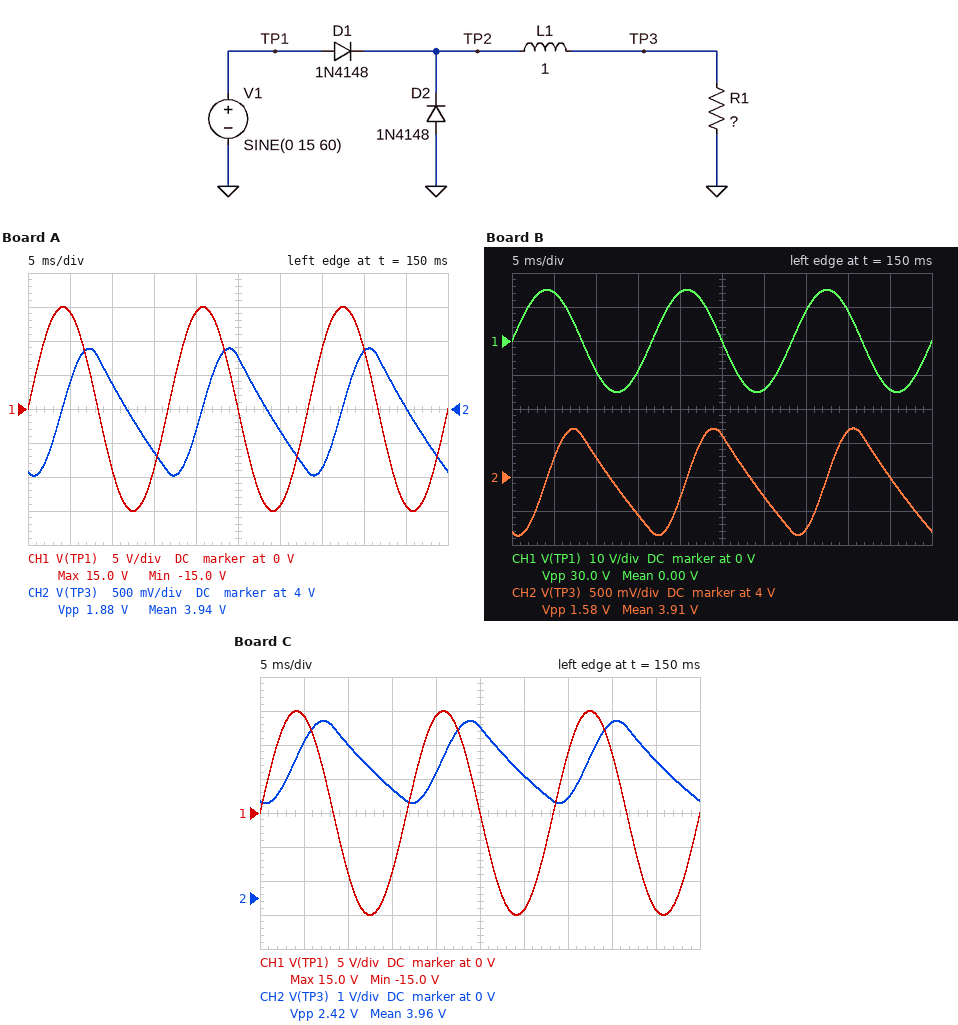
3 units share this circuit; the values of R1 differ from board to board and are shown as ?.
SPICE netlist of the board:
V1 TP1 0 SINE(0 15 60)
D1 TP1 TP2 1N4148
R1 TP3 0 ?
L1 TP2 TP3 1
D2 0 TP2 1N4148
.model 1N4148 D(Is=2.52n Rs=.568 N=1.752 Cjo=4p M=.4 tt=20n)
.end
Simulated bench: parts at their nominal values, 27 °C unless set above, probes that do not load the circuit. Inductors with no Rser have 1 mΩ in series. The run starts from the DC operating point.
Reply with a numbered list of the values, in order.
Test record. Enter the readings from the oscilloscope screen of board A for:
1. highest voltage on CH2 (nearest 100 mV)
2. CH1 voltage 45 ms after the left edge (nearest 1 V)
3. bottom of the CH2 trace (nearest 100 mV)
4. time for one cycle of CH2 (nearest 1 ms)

1. 4.9 V
2. -14 V
3. 3.0 V
4. 17 ms
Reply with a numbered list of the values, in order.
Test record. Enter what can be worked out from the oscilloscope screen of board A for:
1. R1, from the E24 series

1. 43 Ω
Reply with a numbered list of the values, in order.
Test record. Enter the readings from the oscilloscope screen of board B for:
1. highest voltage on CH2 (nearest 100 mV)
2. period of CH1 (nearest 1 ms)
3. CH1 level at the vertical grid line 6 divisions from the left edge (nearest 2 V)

1. 4.7 V
2. 17 ms
3. -14 V
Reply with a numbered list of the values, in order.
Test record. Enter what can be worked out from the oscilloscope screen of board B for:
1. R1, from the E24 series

1. 36 Ω
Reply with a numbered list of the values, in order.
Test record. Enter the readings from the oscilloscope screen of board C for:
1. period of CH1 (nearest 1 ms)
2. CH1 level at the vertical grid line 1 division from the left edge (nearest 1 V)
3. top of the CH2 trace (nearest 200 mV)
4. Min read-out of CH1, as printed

1. 17 ms
2. 14 V
3. 5.2 V
4. -15.0 V
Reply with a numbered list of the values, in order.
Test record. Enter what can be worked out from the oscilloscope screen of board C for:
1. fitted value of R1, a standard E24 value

1. 56 Ω
